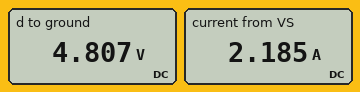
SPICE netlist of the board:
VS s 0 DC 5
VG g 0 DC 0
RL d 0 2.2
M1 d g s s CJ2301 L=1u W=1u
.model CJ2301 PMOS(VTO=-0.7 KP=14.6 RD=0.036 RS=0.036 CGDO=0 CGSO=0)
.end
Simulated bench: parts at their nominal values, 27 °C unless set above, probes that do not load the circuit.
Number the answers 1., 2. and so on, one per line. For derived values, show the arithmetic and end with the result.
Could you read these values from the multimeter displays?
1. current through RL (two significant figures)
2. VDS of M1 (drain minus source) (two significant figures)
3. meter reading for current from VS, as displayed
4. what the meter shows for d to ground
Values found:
1. (4.807 V) / 2.2 Ω = 2.2 A
2. 4.807 V - 5 V = -190 mV
3. 2.185 A
4. 4.807 V
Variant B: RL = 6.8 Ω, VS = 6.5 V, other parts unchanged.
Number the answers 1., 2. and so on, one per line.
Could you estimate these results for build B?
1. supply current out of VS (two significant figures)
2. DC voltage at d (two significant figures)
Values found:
1. 940 mA
2. 6.4 V
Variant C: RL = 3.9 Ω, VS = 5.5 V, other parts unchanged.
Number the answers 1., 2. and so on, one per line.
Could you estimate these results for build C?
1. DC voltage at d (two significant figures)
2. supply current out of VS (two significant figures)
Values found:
1. 5.4 V
2. 1.4 A
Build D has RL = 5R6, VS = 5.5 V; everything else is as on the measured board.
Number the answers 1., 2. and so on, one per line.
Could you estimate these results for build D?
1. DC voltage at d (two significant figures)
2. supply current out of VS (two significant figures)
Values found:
1. 5.4 V
2. 970 mA
